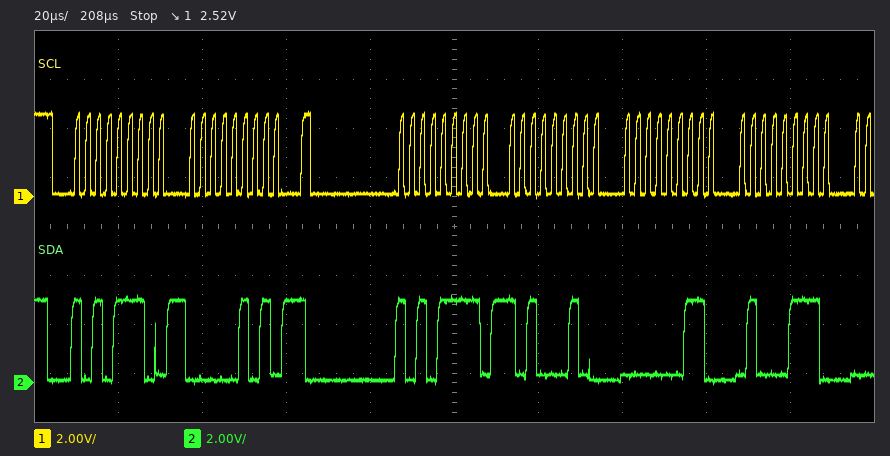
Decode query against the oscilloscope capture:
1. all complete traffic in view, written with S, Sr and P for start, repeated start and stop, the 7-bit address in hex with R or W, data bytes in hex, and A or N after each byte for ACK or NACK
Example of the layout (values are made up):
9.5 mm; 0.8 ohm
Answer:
S 57W A 05 A Sr 57R A A2 A 03 A 47 A
